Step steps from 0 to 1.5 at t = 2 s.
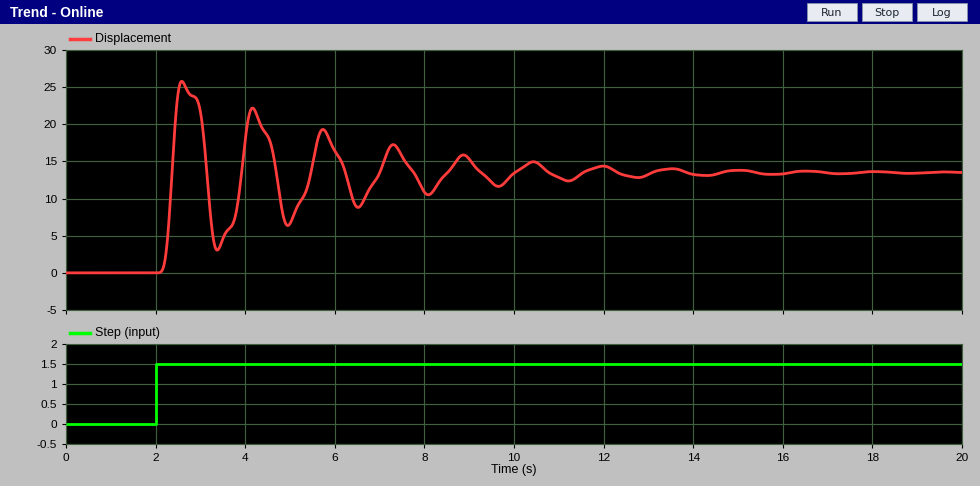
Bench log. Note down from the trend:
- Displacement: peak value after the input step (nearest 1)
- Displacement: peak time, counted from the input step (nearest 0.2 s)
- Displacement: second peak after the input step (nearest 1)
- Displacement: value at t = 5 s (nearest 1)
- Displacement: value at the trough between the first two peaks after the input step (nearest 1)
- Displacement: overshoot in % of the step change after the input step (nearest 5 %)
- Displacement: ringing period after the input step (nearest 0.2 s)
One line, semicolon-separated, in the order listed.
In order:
26; 0.6 s; 22; 7; 3; 90 %; 1.6 s
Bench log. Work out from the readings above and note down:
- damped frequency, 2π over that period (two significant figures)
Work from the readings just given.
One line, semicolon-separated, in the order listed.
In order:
3.9 rad/s
